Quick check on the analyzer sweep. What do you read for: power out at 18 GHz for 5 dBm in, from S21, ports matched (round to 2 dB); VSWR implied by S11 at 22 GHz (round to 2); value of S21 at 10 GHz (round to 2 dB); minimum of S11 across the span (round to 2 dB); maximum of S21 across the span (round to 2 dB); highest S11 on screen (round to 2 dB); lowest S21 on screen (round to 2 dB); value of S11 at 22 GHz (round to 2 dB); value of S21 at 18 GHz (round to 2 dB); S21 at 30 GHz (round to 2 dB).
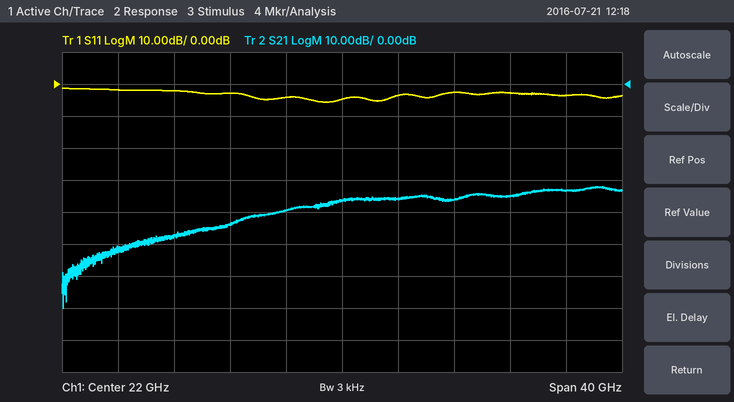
-34 dBm
4
-48 dB
-6 dB
-32 dB
-2 dB
-70 dB
-4 dB
-40 dB
-36 dB
